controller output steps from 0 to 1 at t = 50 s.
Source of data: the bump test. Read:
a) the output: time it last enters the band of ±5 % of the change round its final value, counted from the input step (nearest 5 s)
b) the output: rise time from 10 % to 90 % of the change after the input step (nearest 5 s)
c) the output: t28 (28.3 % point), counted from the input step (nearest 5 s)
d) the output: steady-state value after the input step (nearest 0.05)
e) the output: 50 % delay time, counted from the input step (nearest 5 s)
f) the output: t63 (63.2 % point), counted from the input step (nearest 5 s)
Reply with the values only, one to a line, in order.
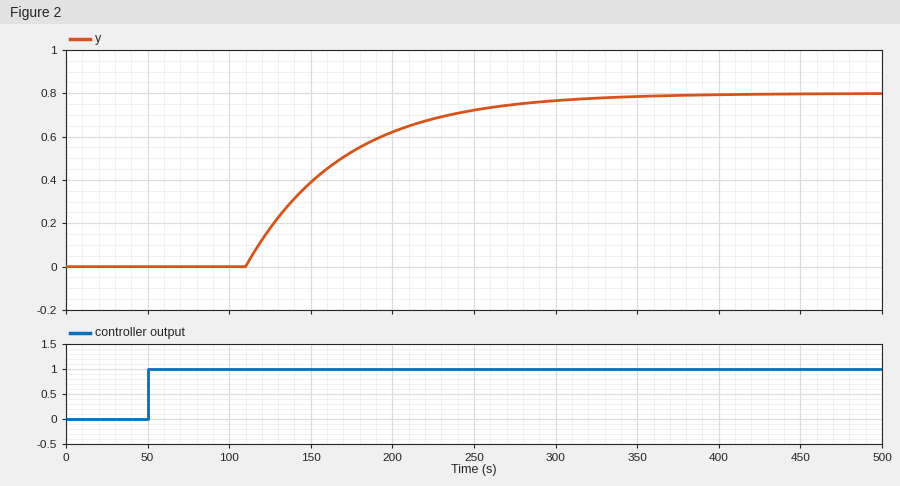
240 s
130 s
80 s
0.80
100 s
120 s
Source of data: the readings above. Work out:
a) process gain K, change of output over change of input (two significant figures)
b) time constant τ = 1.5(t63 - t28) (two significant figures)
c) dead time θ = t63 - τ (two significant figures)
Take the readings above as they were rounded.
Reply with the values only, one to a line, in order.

0.80
60 s
60 s
